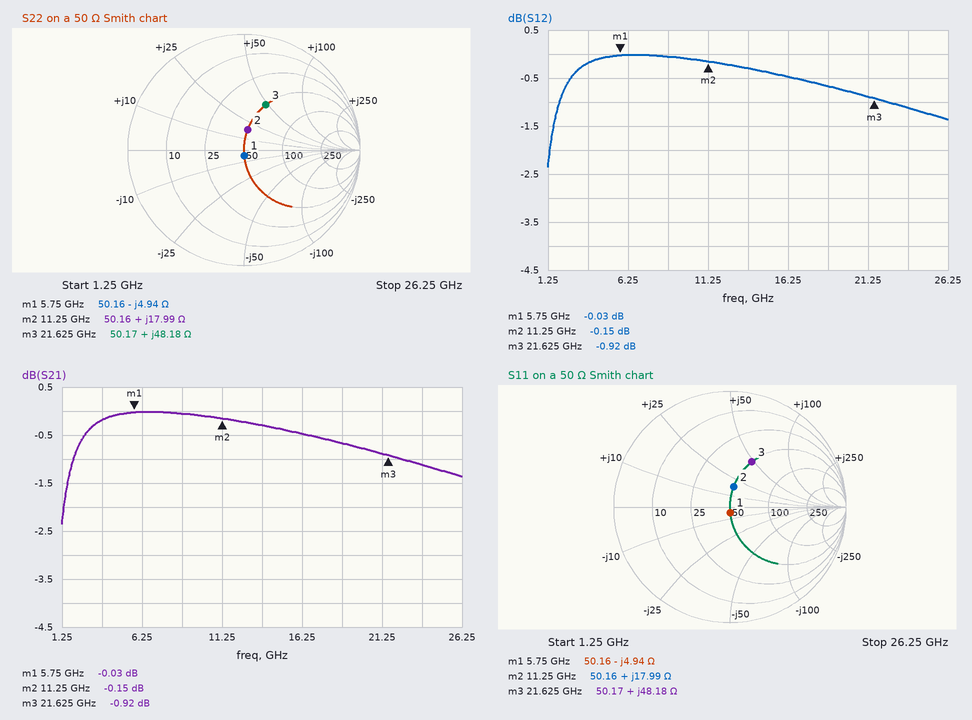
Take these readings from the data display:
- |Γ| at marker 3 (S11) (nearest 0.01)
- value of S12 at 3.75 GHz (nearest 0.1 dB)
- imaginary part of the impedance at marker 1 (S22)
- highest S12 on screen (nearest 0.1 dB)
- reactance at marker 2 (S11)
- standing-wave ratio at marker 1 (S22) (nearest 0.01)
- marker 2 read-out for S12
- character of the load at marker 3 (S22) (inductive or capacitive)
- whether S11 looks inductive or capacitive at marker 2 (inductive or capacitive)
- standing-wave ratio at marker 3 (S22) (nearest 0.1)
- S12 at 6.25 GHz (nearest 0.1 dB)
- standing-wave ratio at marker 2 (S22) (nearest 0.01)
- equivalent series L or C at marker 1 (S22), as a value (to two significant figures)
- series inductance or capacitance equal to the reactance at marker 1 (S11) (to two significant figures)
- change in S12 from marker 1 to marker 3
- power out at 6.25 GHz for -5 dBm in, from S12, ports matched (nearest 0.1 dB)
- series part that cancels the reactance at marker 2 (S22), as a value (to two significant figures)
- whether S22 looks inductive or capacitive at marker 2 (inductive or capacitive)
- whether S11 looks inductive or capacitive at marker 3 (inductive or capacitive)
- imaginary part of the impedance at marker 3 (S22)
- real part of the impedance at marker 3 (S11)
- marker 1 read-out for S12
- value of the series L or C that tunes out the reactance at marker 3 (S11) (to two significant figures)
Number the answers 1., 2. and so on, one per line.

1. 0.43
2. -0.2 dB
3. -4.94 Ω
4. 0.0 dB
5. +17.99 Ω
6. 1.10
7. -0.15 dB
8. inductive
9. inductive
10. 2.5
11. 0.0 dB
12. 1.43
13. 5.6 pF
14. 5.6 pF
15. -0.89 dB
16. -5.0 dBm
17. 790 fF
18. inductive
19. inductive
20. +48.18 Ω
21. 50.17 Ω
22. -0.03 dB
23. 150 fF
